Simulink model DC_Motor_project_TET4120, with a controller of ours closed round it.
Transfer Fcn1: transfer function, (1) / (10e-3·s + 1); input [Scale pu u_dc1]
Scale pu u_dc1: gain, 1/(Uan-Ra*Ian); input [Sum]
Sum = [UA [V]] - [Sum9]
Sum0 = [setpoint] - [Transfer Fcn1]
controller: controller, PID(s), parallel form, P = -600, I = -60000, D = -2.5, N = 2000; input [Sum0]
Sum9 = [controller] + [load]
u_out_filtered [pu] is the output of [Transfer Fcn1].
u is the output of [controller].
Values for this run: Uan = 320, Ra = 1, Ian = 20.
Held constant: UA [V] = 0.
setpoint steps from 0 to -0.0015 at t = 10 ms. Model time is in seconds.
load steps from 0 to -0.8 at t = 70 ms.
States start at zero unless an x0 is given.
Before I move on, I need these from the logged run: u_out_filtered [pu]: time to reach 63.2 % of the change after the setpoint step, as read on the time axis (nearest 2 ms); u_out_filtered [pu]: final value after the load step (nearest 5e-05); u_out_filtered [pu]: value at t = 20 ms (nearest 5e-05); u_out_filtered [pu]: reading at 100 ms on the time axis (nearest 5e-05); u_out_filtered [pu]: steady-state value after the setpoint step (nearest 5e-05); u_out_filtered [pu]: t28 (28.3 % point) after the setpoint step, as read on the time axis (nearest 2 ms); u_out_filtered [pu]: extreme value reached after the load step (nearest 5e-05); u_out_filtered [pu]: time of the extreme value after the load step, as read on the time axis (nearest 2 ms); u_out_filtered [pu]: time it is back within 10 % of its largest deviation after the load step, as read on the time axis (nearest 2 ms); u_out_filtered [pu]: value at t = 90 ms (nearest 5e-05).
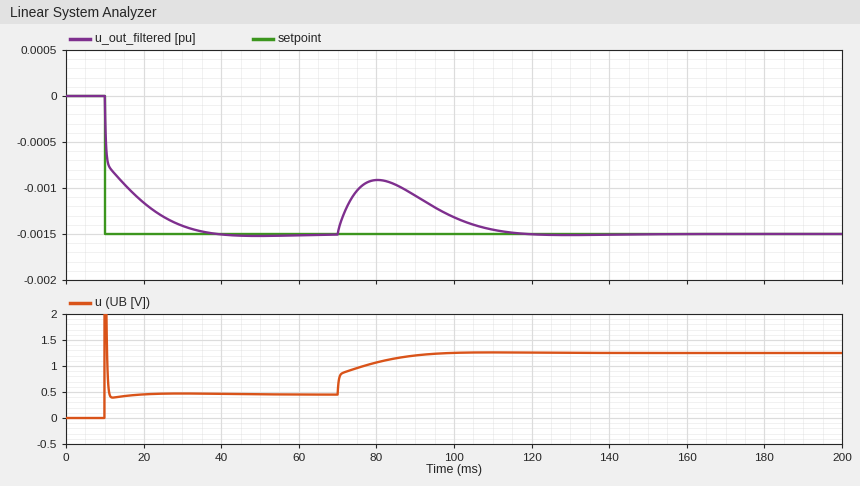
14 ms
-0.00150
-0.00115
-0.00130
-0.00150
10 ms
-0.00090
80 ms
108 ms
-0.00110
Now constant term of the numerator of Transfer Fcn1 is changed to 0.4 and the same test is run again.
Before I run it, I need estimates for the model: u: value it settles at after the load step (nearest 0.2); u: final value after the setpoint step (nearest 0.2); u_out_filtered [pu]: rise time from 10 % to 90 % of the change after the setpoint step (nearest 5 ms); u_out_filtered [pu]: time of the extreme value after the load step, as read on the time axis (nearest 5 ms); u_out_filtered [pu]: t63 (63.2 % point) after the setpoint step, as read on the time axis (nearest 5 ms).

2.0
1.2
30 ms
85 ms
25 ms
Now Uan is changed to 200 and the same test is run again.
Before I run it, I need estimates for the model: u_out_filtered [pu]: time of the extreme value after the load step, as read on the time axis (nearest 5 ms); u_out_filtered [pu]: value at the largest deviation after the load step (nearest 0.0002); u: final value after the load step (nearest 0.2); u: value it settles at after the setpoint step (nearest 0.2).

80 ms
-0.0008
1.0
0.2
